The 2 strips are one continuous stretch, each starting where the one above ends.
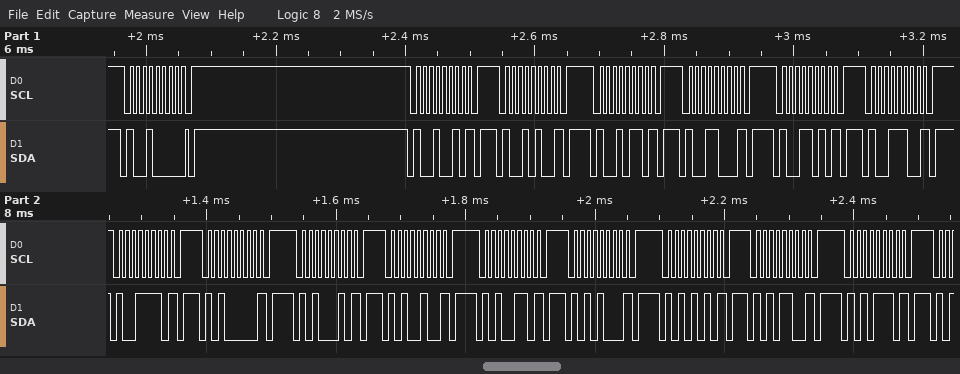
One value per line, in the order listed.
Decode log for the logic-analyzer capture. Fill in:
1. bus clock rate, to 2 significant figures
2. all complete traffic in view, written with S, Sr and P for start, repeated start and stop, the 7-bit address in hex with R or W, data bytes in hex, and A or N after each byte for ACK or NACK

100 kHz
S 48W A P S 49W N P S 4AW N P S 4BW N P S 4CW N P S 4DW N P S 4EW N P S 4FW N P S 50W N P S 51W N P S 52W N P S 53W N P S 54W N P S 55W N P S 56W N P S 57W N P
